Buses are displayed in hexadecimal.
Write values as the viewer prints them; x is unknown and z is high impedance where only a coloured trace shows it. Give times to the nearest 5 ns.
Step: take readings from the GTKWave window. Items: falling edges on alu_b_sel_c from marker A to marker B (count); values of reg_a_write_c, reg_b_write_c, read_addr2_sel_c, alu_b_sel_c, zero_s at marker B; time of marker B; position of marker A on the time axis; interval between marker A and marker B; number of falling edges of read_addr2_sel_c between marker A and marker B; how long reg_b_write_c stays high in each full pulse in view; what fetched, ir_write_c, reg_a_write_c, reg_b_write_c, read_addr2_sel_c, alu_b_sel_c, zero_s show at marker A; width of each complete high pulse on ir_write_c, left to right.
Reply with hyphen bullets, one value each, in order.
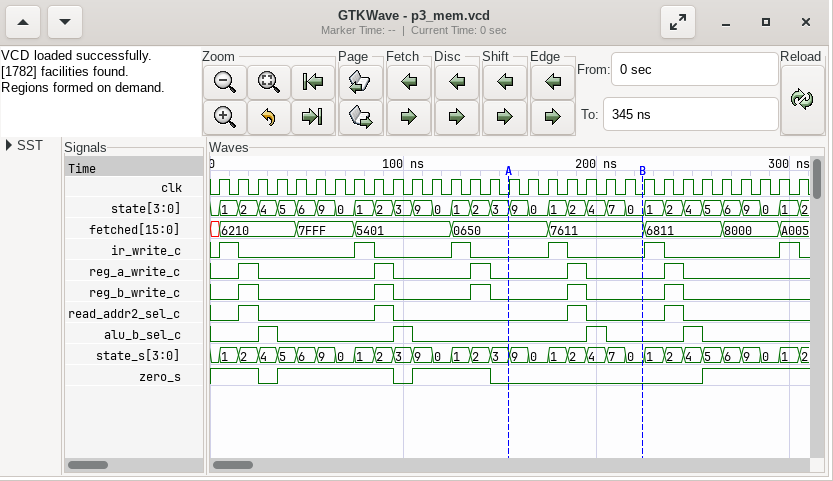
- 1
- reg_a_write_c=0, reg_b_write_c=0, read_addr2_sel_c=0, alu_b_sel_c=0, zero_s=0
- 225 ns
- 155 ns
- 70 ns
- 1
- 10 ns, 10 ns, 10 ns, 10 ns, 10 ns
- fetched=0650, ir_write_c=0, reg_a_write_c=0, reg_b_write_c=0, read_addr2_sel_c=0, alu_b_sel_c=0, zero_s=0
- 10 ns, 10 ns, 10 ns, 10 ns, 10 ns, 10 ns
